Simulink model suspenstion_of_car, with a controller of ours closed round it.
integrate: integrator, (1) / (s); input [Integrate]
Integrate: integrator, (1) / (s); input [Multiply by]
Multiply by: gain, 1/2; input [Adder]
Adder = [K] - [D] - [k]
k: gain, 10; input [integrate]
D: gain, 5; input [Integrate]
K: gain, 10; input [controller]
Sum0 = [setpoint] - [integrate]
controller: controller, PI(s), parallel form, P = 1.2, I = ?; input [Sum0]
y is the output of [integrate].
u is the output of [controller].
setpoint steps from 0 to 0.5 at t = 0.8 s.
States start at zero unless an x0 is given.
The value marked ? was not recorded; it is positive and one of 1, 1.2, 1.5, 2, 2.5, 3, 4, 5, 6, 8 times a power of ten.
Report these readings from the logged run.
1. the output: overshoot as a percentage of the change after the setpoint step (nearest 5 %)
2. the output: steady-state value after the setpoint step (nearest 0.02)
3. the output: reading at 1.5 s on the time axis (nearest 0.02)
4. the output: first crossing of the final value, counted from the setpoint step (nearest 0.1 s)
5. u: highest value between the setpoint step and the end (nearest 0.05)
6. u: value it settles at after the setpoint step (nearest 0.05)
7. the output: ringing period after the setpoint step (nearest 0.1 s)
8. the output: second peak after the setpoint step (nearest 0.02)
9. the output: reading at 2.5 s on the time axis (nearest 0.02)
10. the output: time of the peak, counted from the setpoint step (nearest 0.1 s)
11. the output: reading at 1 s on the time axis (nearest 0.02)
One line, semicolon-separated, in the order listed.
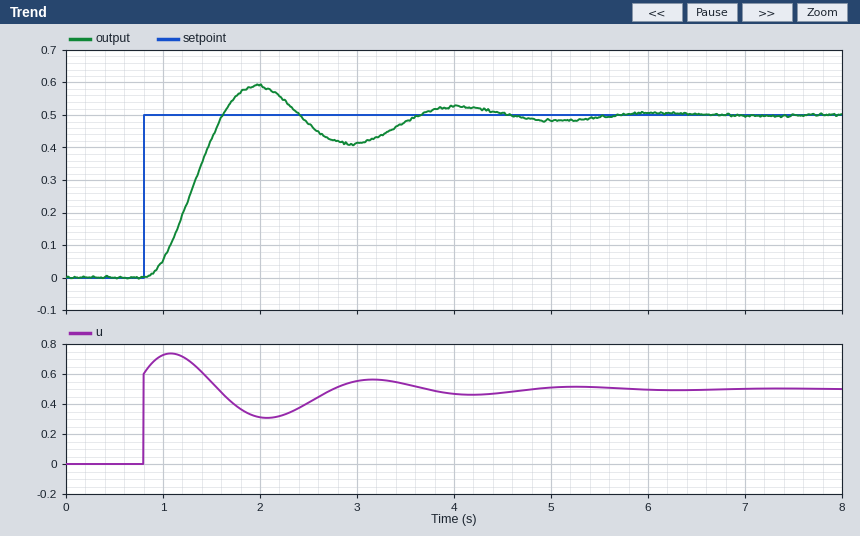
20 %; 0.50; 0.42; 0.8 s; 0.75; 0.50; 2.1 s; 0.52; 0.48; 1.2 s; 0.06
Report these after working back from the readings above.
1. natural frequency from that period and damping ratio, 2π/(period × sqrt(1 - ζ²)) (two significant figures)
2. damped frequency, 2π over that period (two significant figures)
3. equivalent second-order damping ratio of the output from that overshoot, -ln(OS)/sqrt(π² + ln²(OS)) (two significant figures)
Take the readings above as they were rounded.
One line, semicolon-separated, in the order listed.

3.4 rad/s; 3.0 rad/s; 0.46
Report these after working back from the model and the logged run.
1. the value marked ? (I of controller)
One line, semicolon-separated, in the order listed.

2
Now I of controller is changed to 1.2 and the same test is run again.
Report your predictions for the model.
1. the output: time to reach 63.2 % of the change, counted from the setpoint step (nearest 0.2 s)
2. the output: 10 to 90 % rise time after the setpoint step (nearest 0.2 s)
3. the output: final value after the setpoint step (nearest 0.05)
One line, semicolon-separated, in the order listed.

0.6 s; 0.6 s; 0.50
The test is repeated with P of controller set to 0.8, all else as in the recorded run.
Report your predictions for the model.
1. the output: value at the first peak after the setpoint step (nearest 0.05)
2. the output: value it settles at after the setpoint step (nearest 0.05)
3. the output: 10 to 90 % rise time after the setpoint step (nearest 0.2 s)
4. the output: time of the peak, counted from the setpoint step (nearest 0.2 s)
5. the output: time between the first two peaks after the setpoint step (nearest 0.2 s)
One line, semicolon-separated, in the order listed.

0.60; 0.50; 0.6 s; 1.4 s; 2.4 s
